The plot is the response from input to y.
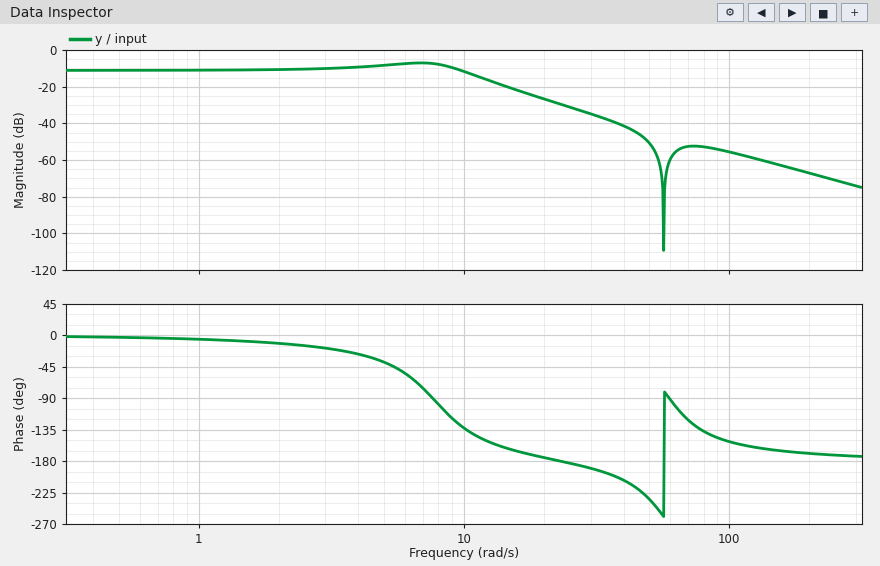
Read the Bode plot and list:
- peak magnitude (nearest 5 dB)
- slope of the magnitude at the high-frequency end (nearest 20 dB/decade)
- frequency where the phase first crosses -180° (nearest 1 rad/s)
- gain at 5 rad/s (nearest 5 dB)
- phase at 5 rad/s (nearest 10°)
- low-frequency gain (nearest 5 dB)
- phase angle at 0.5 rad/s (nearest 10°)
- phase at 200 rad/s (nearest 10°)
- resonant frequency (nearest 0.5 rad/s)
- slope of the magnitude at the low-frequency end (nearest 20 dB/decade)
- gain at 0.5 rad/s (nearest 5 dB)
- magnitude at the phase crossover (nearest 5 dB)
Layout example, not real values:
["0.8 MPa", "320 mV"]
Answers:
["-5 dB", "-40 dB/decade", "23 rad/s", "-10 dB", "-40°", "-10 dB", "0°", "-170°", "7.0 rad/s", "0 dB/decade", "-10 dB", "-30 dB"]
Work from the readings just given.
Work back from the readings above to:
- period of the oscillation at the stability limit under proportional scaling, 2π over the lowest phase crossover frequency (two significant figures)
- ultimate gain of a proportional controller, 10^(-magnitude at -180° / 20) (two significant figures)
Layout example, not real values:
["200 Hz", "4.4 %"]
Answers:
["0.27 s", "32"]
